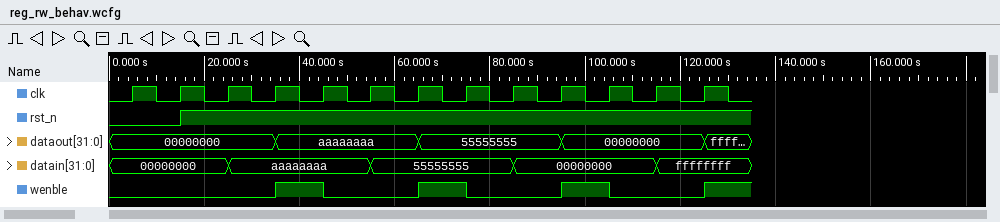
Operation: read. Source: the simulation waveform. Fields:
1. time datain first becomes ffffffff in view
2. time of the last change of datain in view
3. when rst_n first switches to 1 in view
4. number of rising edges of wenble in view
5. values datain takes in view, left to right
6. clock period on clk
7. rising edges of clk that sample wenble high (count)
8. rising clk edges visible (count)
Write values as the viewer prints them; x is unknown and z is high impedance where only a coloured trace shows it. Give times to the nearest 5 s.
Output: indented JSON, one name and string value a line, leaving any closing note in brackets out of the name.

{
  "time datain first becomes ffffffff in view": "115 s",
  "time of the last change of datain in view": "115 s",
  "when rst_n first switches to 1 in view": "15 s",
  "number of rising edges of wenble in view": "4",
  "values datain takes in view, left to right": "00000000, aaaaaaaa, 55555555, 00000000, ffffffff",
  "clock period on clk": "10 s",
  "rising edges of clk that sample wenble high": "3",
  "rising clk edges visible": "13"
}
